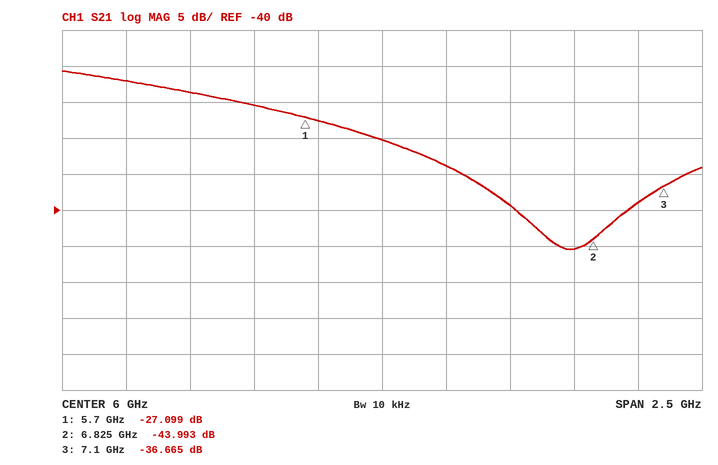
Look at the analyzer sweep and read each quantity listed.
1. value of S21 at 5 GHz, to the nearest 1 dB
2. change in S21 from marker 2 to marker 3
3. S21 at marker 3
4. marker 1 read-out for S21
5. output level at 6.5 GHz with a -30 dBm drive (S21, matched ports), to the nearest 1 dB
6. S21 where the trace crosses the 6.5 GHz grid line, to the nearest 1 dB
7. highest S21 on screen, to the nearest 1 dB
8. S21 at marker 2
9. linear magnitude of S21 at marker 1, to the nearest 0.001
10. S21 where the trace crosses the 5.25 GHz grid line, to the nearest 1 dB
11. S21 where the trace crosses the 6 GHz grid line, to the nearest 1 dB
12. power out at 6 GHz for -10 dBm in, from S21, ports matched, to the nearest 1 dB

-22 dB
7.328 dB
-36.665 dB
-27.099 dB
-69 dBm
-39 dB
-21 dB
-43.993 dB
0.044
-24 dB
-30 dB
-40 dBm
